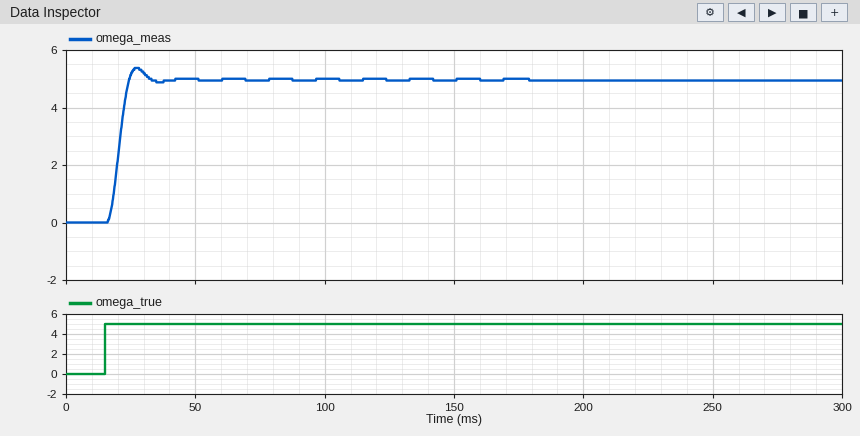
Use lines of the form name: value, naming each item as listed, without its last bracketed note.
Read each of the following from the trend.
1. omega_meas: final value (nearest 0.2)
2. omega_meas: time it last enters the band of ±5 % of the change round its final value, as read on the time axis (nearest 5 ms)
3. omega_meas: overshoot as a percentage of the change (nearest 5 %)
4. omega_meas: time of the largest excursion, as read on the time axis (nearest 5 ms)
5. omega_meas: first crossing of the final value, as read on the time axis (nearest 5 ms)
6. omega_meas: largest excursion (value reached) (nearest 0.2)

omega_meas: final value: 5.0
omega_meas: time it last enters the band of ±5 % of the change round its final value, as read on the time axis: 30 ms
omega_meas: overshoot as a percentage of the change: 10 %
omega_meas: time of the largest excursion, as read on the time axis: 25 ms
omega_meas: first crossing of the final value, as read on the time axis: 25 ms
omega_meas: largest excursion (value reached): 5.4
